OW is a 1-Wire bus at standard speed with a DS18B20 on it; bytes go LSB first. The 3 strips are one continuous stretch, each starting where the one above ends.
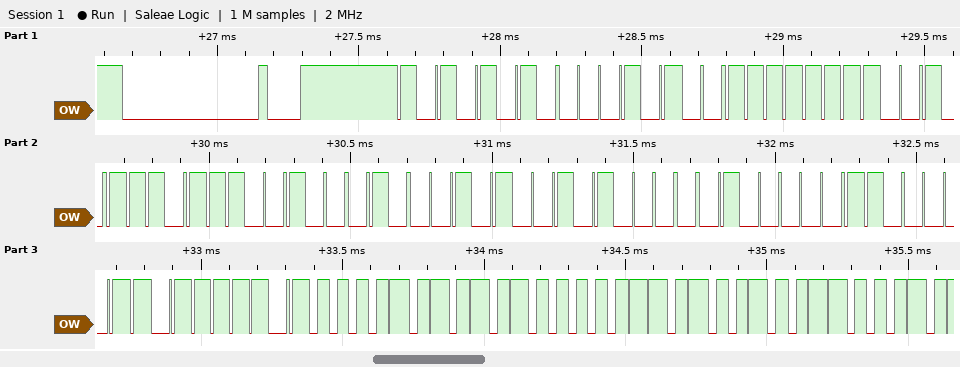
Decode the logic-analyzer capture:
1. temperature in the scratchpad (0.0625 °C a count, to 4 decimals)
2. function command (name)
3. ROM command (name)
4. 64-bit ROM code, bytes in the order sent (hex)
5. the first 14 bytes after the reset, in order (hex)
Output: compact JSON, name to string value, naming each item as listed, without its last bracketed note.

{"temperature in the scratchpad": "85.0000 °C", "function command": "Read Scratchpad", "ROM command": "Match ROM", "64-bit ROM code, bytes in the order sent": "28 FF 74 27 A2 14 04 C3", "the first 14 bytes after the reset, in order": "55 28 FF 74 27 A2 14 04 C3 BE 50 05 4B 46"}
